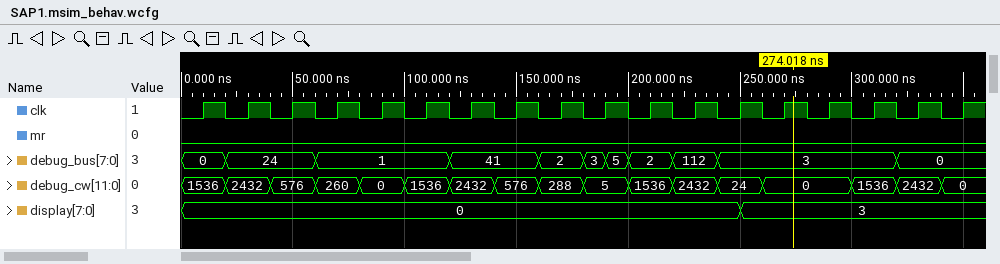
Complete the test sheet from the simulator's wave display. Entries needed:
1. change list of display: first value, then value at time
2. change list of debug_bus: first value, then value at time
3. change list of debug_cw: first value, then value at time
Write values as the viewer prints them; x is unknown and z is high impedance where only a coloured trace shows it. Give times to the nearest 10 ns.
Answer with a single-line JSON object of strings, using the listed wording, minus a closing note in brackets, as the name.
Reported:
{"change list of display: first value, then value at time": "0, 3 at 250 ns", "change list of debug_bus: first value, then value at time": "0, 24 at 20 ns, 1 at 60 ns, 41 at 120 ns, 2 at 160 ns, 3 at 180 ns, 5 at 190 ns, 2 at 200 ns, 112 at 220 ns, 3 at 240 ns, 0 at 320 ns", "change list of debug_cw: first value, then value at time": "1536, 2432 at 20 ns, 576 at 40 ns, 260 at 60 ns, 0 at 80 ns, 1536 at 100 ns, 2432 at 120 ns, 576 at 140 ns, 288 at 160 ns, 5 at 180 ns, 1536 at 200 ns, 2432 at 220 ns, 24 at 240 ns, 0 at 260 ns, 1536 at 300 ns, 2432 at 320 ns, 0 at 340 ns"}
